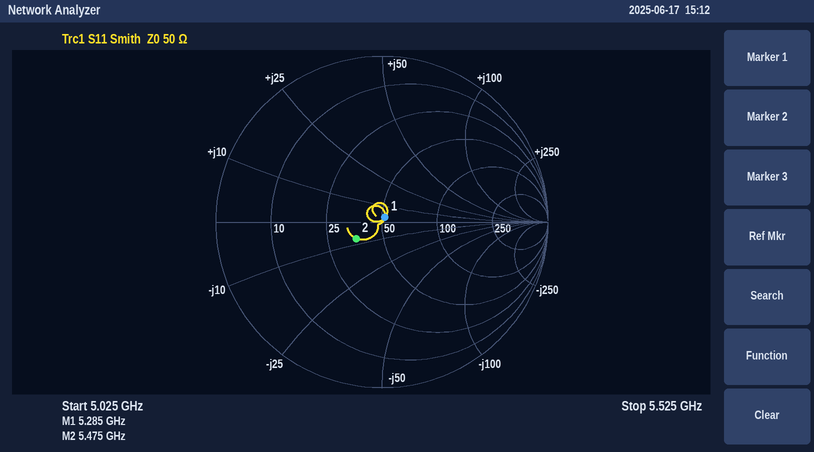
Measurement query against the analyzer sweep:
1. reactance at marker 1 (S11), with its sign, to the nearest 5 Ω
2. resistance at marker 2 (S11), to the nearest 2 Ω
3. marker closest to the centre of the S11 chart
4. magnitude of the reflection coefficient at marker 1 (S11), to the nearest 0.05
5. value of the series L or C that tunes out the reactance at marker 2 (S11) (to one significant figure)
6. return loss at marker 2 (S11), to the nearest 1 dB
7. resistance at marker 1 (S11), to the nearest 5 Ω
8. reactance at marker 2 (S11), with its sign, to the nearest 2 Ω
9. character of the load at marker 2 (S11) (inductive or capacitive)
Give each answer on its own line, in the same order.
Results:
+5 Ω
36 Ω
marker 1
0.05
200 pH
15 dB
50 Ω
-8 Ω
capacitive
